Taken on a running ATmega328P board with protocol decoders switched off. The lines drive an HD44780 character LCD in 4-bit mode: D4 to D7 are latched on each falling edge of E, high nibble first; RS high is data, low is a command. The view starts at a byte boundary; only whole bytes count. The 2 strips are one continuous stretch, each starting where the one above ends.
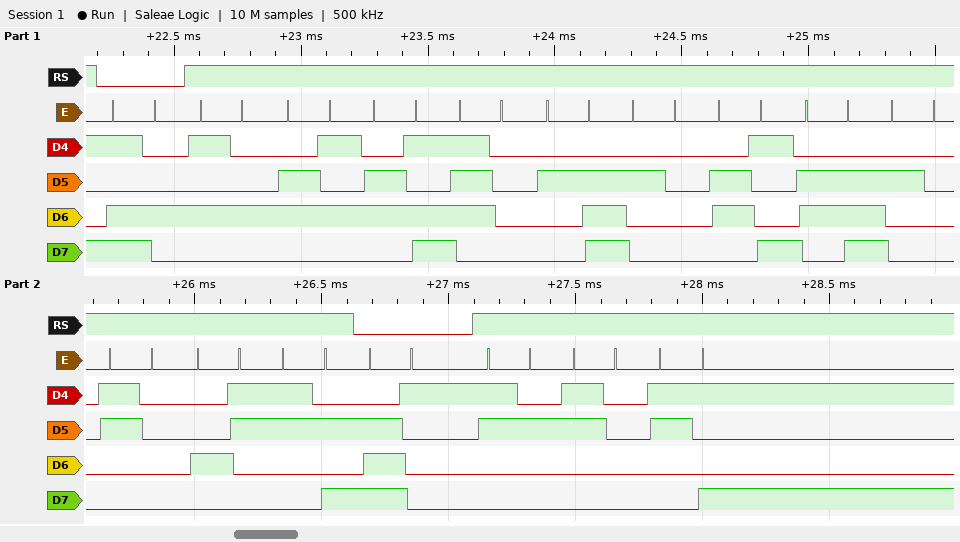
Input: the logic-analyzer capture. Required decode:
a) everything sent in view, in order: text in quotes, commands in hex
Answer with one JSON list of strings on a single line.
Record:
["0xD4 \"Temp. in 0C:\" 0xE1 \"209\""]
